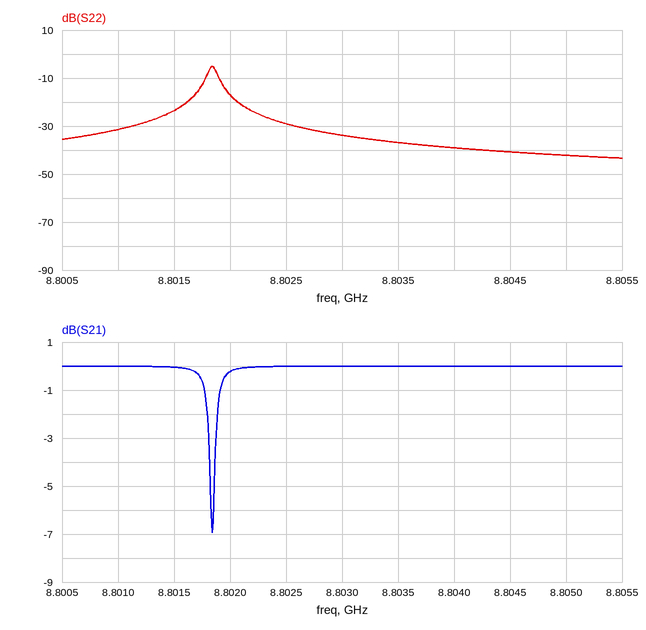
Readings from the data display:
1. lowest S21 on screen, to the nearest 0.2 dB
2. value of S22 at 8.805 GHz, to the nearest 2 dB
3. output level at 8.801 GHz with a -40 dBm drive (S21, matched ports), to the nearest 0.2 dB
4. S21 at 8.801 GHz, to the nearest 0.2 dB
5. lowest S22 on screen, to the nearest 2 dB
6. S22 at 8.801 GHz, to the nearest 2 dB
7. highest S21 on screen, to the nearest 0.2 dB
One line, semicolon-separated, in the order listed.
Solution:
-7.0 dB; -42 dB; -40.0 dBm; 0.0 dB; -44 dB; -32 dB; 0.0 dB
